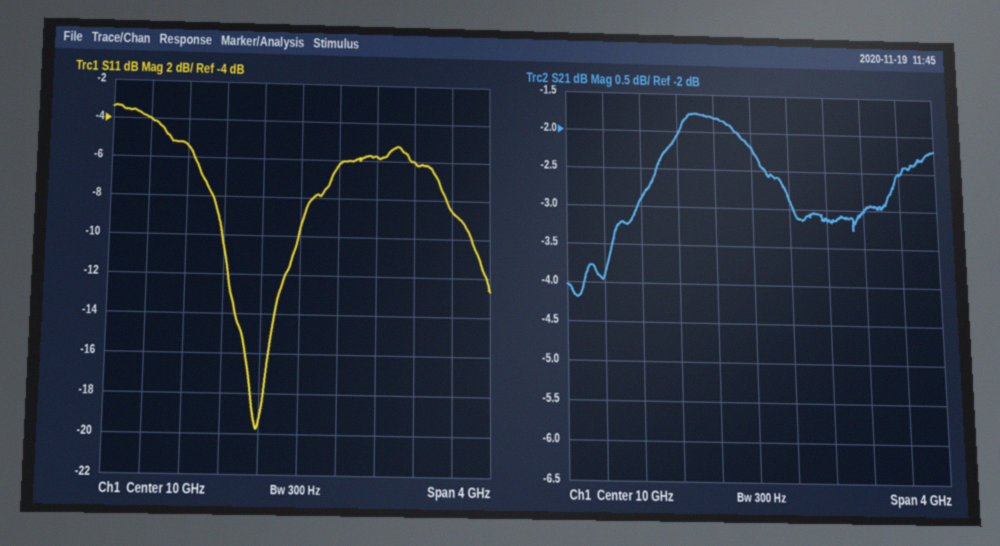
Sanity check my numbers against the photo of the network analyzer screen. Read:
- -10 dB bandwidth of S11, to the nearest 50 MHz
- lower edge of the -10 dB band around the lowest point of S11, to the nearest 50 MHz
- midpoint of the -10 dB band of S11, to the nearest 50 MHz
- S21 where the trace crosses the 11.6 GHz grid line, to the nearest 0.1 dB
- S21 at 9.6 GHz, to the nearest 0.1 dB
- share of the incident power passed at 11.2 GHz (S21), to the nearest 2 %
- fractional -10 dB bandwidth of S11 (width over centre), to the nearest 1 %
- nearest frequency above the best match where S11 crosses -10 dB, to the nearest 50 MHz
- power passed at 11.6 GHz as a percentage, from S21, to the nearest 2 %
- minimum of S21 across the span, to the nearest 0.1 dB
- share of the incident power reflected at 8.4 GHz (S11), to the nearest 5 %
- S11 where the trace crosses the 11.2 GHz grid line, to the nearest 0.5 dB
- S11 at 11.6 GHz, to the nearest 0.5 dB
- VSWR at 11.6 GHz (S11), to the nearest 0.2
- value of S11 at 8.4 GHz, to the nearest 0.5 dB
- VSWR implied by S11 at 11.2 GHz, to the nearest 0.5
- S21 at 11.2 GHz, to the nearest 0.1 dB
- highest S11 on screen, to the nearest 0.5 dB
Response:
800 MHz
9.20 GHz
9.60 GHz
-2.5 dB
-1.8 dB
50 %
8 %
10.00 GHz
56 %
-4.2 dB
40 %
-6.0 dB
-8.5 dB
2.2
-4.0 dB
3.0
-3.0 dB
-3.5 dB
